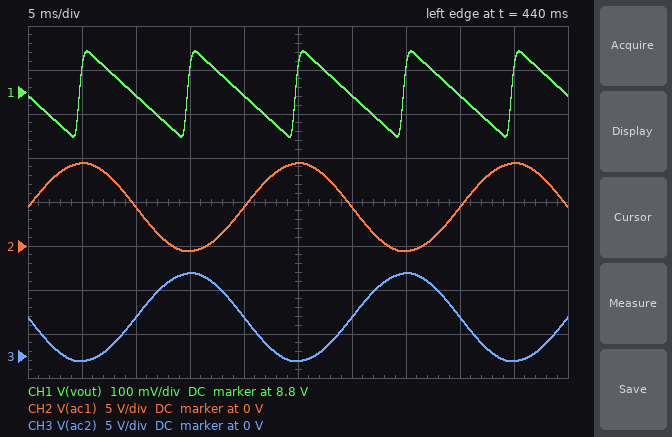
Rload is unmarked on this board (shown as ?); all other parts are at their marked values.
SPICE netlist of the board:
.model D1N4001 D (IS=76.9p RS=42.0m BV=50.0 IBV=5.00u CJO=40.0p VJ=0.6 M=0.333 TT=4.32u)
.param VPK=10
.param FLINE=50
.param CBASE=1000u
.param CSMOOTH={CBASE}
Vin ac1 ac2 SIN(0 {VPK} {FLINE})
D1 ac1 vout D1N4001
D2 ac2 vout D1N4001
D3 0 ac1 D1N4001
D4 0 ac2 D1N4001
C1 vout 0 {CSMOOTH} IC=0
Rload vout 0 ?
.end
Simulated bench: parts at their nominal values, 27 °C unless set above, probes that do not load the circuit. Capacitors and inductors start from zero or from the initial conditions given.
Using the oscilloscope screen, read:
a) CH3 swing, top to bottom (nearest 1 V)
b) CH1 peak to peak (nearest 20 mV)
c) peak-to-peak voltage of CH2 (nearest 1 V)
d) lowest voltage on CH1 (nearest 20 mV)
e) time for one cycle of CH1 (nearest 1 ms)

10 V
200 mV
10 V
8.70 V
10 ms
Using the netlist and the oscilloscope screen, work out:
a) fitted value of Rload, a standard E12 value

390 Ω
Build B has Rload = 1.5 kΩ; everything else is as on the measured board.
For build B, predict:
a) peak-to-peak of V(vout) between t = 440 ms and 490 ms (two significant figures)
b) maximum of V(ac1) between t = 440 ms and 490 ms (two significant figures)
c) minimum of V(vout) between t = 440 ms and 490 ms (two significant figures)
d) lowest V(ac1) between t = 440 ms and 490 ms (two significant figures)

52 mV
9.5 V
8.9 V
-550 mV
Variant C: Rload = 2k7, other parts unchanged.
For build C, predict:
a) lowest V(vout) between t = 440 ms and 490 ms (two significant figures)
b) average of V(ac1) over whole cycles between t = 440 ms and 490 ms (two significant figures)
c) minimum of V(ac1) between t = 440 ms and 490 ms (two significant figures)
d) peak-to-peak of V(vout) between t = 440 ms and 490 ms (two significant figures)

8.9 V
4.5 V
-530 mV
29 mV
